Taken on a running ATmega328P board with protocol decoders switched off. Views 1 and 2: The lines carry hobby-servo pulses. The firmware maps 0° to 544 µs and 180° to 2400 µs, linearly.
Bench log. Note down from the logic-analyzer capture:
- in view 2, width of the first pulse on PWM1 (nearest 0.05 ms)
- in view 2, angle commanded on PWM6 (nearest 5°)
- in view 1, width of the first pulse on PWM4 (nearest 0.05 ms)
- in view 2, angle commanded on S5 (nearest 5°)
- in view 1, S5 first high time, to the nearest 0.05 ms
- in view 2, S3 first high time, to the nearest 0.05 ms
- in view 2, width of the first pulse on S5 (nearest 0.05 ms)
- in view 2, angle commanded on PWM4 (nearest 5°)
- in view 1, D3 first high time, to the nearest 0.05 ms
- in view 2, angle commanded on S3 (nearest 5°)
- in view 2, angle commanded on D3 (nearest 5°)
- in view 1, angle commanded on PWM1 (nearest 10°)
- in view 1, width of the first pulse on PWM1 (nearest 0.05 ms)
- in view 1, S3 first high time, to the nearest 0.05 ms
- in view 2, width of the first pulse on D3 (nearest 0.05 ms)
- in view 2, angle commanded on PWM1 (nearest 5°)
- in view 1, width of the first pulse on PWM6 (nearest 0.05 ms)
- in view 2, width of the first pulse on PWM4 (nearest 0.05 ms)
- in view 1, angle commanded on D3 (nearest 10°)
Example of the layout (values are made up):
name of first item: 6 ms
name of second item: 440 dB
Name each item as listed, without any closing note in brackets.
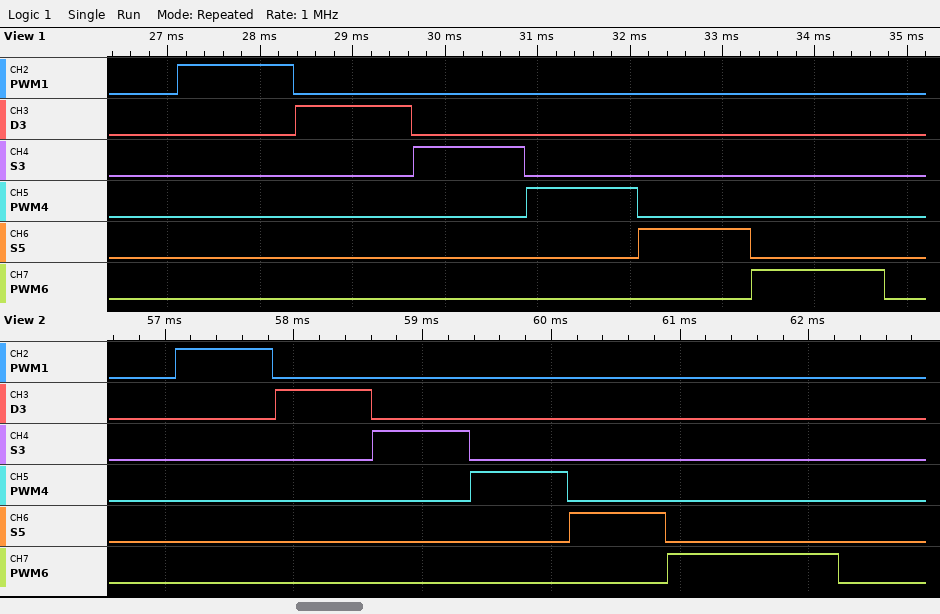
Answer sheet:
in view 2, width of the first pulse on PWM1: 0.75 ms
in view 2, angle commanded on PWM6: 75°
in view 1, width of the first pulse on PWM4: 1.20 ms
in view 2, angle commanded on S5: 20°
in view 1, S5 first high time, to the nearest 0.05 ms: 1.20 ms
in view 2, S3 first high time, to the nearest 0.05 ms: 0.75 ms
in view 2, width of the first pulse on S5: 0.75 ms
in view 2, angle commanded on PWM4: 20°
in view 1, D3 first high time, to the nearest 0.05 ms: 1.25 ms
in view 2, angle commanded on S3: 20°
in view 2, angle commanded on D3: 20°
in view 1, angle commanded on PWM1: 70°
in view 1, width of the first pulse on PWM1: 1.25 ms
in view 1, S3 first high time, to the nearest 0.05 ms: 1.20 ms
in view 2, width of the first pulse on D3: 0.75 ms
in view 2, angle commanded on PWM1: 20°
in view 1, width of the first pulse on PWM6: 1.45 ms
in view 2, width of the first pulse on PWM4: 0.75 ms
in view 1, angle commanded on D3: 70°
